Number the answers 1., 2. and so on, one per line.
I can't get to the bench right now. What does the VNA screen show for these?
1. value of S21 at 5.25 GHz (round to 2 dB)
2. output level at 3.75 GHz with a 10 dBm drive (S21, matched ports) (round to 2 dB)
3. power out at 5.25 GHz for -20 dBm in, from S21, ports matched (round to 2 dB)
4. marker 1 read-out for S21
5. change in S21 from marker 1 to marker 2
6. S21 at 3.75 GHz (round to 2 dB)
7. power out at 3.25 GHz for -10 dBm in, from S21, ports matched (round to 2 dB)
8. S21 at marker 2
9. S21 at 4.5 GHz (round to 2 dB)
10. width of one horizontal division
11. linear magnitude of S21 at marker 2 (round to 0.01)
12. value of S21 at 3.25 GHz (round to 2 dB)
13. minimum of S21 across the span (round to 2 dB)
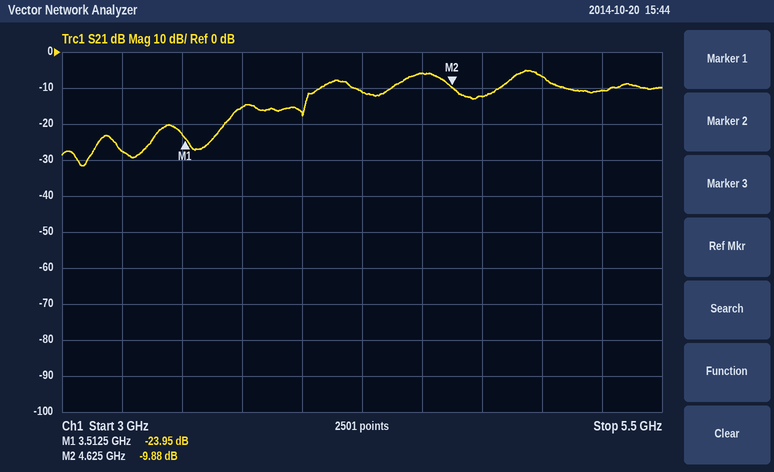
1. -10 dB
2. -6 dBm
3. -30 dBm
4. -23.95 dB
5. 14.07 dB
6. -16 dB
7. -38 dBm
8. -9.88 dB
9. -6 dB
10. 250 MHz
11. 0.32
12. -28 dB
13. -32 dB
